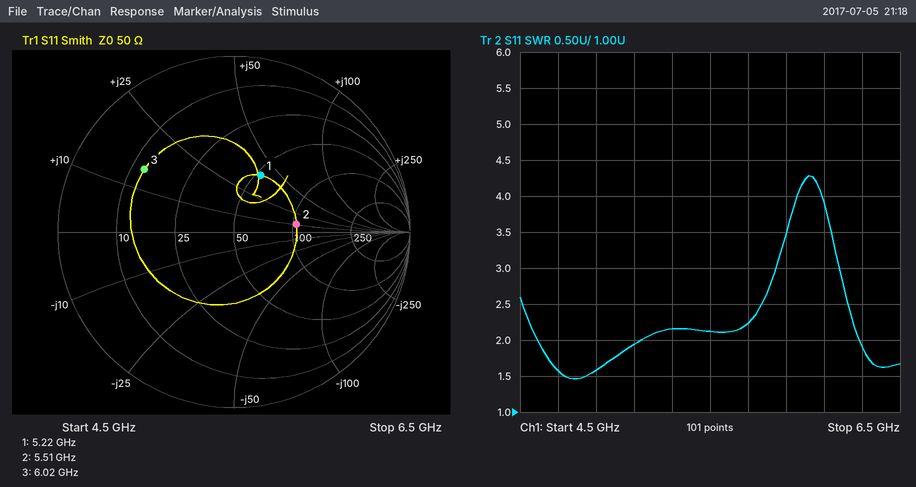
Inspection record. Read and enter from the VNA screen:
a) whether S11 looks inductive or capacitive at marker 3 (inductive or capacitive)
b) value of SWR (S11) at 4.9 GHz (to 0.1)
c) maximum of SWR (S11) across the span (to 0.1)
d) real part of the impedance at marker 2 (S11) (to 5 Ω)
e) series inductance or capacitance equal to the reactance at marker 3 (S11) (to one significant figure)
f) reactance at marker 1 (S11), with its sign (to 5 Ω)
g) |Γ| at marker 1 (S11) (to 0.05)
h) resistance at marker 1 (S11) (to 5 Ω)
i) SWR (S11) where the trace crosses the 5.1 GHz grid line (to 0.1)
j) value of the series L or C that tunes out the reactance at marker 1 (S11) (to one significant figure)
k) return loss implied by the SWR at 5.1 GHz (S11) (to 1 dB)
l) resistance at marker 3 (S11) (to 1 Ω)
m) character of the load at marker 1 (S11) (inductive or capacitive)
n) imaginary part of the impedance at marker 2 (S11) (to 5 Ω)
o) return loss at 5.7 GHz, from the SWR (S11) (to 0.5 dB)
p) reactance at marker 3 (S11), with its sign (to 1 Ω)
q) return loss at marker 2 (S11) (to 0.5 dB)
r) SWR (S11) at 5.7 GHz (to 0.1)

inductive
1.6
4.3
105 Ω
400 pH
+40 Ω
0.35
55 Ω
1.9
800 fF
10 dB
13 Ω
inductive
+10 Ω
8.5 dB
+15 Ω
9.0 dB
2.2
